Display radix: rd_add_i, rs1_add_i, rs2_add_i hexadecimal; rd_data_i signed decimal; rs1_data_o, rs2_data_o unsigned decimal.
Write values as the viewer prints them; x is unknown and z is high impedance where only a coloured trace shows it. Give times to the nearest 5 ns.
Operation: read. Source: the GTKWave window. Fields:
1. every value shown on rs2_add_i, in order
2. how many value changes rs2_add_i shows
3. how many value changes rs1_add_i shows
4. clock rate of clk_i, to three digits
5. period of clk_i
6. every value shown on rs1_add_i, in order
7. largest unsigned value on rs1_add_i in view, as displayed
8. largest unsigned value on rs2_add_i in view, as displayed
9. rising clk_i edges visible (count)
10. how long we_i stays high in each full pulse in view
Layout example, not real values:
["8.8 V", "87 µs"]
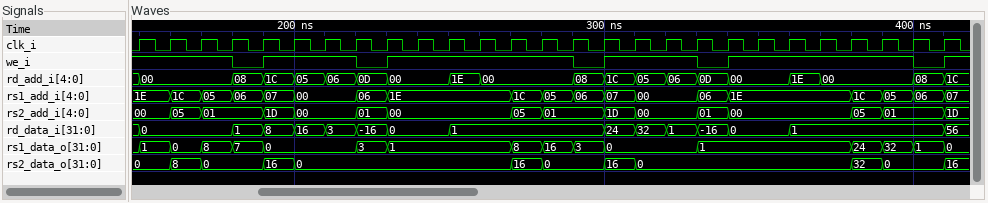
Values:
["00, 05, 01, 1D, 00, 01, 00, 05, 01, 1D, 00, 01, 00, 05, 01, 1D", "15", "18", "100 MHz", "10 ns", "1E, 1C, 05, 06, 07, 00, 06, 1E, 1C, 05, 06, 07, 00, 06, 1E, 1C, 05, 06, 07", "1E", "1D", "27", "30 ns, 60 ns, 30 ns, 60 ns"]
